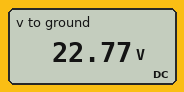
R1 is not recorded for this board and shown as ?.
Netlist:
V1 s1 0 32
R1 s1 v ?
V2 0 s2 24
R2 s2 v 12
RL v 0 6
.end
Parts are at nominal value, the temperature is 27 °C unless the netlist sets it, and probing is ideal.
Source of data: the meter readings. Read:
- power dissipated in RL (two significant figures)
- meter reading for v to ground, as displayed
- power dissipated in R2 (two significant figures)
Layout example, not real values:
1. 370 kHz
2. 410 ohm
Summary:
1. 86 W
2. 22.77 V
3. 180 W
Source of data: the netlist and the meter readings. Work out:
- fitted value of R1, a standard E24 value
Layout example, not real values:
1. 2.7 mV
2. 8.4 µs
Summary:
1. 1.2 Ω
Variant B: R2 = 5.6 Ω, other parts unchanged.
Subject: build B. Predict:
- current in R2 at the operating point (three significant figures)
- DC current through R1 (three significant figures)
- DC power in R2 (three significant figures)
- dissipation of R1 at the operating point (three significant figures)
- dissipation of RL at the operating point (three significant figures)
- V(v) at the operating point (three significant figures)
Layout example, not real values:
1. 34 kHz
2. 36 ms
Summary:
1. 7.68 A
2. 10.8 A
3. 330 W
4. 141 W
5. 60.1 W
6. 19.0 V
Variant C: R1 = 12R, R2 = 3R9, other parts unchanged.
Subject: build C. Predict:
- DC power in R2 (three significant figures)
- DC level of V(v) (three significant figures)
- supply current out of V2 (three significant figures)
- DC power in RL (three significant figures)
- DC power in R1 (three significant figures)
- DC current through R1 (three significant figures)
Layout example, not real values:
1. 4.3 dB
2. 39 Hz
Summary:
1. 75.1 W
2. -6.89 V
3. 4.39 A
4. 7.90 W
5. 126 W
6. 3.24 A
